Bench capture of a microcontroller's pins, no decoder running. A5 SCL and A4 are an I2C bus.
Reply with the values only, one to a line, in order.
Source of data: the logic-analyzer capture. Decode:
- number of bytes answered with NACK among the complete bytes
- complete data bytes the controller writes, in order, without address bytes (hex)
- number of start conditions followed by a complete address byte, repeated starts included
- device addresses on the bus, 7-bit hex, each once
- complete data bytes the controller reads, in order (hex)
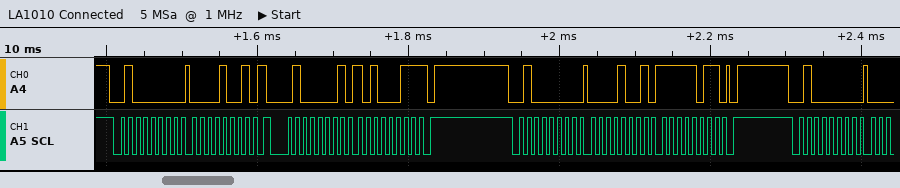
1
09 09 FB
4
0x20
A3
